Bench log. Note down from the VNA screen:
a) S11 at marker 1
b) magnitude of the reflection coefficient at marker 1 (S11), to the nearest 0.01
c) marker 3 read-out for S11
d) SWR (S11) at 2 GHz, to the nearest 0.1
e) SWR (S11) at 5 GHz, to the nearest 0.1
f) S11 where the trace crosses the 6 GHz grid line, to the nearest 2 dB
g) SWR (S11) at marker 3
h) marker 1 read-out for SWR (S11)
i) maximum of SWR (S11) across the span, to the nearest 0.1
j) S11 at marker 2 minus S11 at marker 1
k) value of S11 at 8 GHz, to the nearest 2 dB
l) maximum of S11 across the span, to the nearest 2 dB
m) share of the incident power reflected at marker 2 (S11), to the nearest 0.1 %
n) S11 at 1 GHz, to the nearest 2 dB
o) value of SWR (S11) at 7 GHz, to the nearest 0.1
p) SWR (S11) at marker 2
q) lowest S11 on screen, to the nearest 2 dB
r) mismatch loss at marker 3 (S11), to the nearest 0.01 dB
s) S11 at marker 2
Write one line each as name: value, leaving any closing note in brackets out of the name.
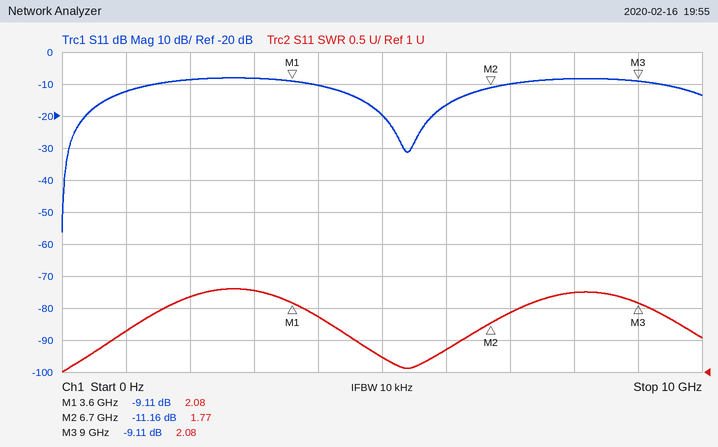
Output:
S11 at marker 1: -9.11 dB
magnitude of the reflection coefficient at marker 1 (S11), to the nearest 0.01: 0.35
marker 3 read-out for S11: -9.11 dB
SWR (S11) at 2 GHz, to the nearest 0.1: 2.2
SWR (S11) at 5 GHz, to the nearest 0.1: 1.2
S11 where the trace crosses the 6 GHz grid line, to the nearest 2 dB: -16 dB
SWR (S11) at marker 3: 2.08
marker 1 read-out for SWR: 2.08
maximum of SWR (S11) across the span, to the nearest 0.1: 2.3
S11 at marker 2 minus S11 at marker 1: -2.05 dB
value of S11 at 8 GHz, to the nearest 2 dB: -8 dB
maximum of S11 across the span, to the nearest 2 dB: -8 dB
share of the incident power reflected at marker 2 (S11), to the nearest 0.1 %: 7.7 %
S11 at 1 GHz, to the nearest 2 dB: -12 dB
value of SWR (S11) at 7 GHz, to the nearest 0.1: 1.9
SWR (S11) at marker 2: 1.77
lowest S11 on screen, to the nearest 2 dB: -56 dB
mismatch loss at marker 3 (S11), to the nearest 0.01 dB: 0.57 dB
S11 at marker 2: -11.16 dB
